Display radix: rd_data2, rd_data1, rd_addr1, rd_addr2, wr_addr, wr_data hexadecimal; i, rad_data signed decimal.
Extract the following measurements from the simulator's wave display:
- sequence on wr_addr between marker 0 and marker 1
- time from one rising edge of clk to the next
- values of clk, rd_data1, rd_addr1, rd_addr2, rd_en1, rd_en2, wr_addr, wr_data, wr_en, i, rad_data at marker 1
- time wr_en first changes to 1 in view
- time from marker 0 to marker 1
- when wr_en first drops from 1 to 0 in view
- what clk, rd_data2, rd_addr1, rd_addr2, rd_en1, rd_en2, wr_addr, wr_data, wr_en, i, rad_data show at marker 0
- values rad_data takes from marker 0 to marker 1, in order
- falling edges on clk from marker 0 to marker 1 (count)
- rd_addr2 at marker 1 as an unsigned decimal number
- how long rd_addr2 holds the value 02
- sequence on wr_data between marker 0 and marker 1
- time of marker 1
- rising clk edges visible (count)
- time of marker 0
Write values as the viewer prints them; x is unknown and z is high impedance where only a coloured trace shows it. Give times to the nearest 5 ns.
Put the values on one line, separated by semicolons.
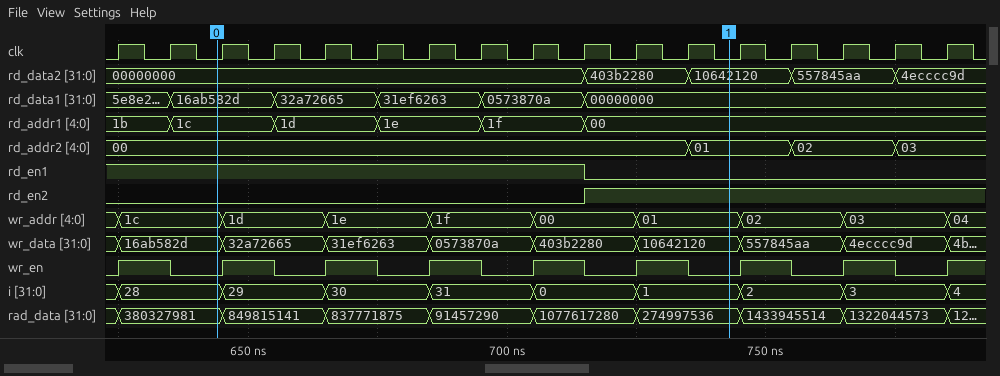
1c, 1d, 1e, 1f, 00, 01; 10 ns; clk=0, rd_data1=00000000, rd_addr1=00, rd_addr2=01, rd_en1=0, rd_en2=1, wr_addr=01, wr_data=10642120, wr_en=0, i=1, rad_data=274997536; 625 ns; 100 ns; 635 ns; clk=0, rd_data2=00000000, rd_addr1=1c, rd_addr2=00, rd_en1=1, rd_en2=0, wr_addr=1c, wr_data=16ab582d, wr_en=0, i=28, rad_data=380327981; 380327981, 849815141, 837771875, 91457290, 1077617280, 274997536; 10; 1; 20 ns; 16ab582d, 32a72665, 31ef6263, 0573870a, 403b2280, 10642120; 745 ns; 17; 645 ns
